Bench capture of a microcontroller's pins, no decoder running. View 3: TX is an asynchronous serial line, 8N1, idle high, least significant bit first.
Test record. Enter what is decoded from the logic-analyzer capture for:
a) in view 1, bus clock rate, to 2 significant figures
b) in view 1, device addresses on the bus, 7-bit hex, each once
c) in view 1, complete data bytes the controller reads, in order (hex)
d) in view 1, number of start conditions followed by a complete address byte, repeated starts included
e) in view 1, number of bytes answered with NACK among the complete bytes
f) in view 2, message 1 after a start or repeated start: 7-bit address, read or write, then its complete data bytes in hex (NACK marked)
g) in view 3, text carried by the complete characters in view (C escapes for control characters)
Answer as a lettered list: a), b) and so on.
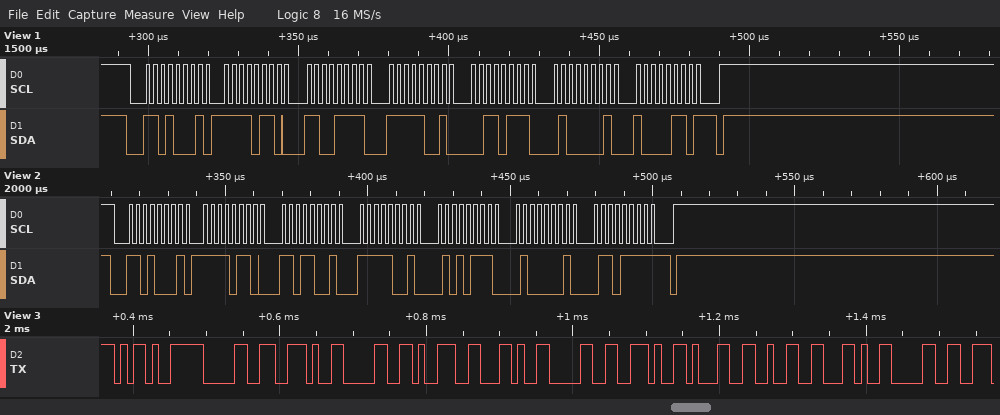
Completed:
a) 400 kHz
b) 0x68
c) F6 CF F9 37 41 86
d) 1
e) 1
f) 0x68 read: F6 D9 F9 57 41 6F NACK
g) "-0.09,0.12,0"
